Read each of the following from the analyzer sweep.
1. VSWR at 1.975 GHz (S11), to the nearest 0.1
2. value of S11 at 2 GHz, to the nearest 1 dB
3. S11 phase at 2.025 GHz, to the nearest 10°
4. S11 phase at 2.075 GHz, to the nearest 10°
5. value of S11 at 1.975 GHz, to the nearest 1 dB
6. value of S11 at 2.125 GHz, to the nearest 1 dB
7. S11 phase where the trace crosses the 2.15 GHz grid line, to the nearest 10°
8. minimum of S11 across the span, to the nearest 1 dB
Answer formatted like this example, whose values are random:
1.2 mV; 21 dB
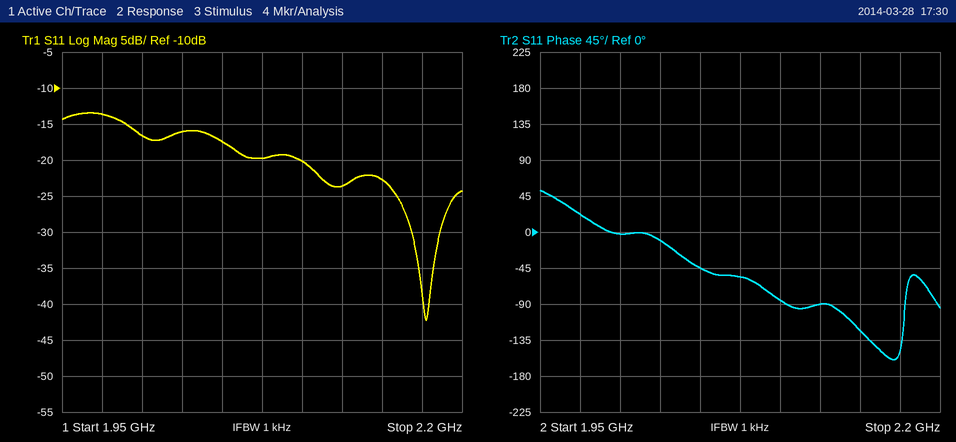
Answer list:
1.5; -17 dB; -10°; -60°; -14 dB; -24 dB; -120°; -42 dB
